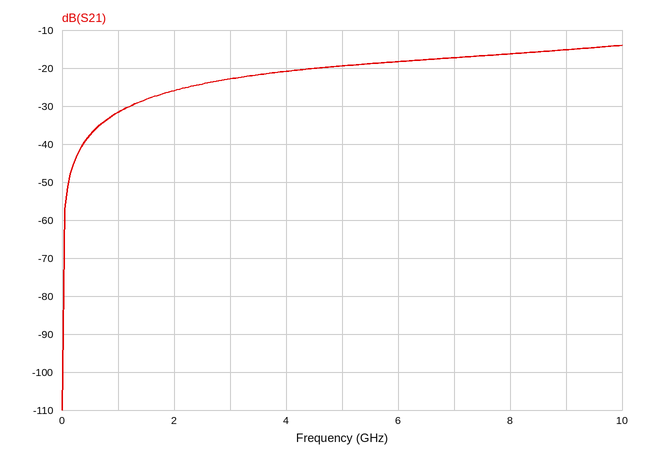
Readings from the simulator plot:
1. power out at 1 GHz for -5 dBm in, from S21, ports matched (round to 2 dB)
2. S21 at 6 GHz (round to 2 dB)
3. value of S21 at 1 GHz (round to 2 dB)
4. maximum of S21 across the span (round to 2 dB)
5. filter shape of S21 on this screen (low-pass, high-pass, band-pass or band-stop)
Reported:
-36 dBm
-18 dB
-32 dB
-14 dB
high-pass
